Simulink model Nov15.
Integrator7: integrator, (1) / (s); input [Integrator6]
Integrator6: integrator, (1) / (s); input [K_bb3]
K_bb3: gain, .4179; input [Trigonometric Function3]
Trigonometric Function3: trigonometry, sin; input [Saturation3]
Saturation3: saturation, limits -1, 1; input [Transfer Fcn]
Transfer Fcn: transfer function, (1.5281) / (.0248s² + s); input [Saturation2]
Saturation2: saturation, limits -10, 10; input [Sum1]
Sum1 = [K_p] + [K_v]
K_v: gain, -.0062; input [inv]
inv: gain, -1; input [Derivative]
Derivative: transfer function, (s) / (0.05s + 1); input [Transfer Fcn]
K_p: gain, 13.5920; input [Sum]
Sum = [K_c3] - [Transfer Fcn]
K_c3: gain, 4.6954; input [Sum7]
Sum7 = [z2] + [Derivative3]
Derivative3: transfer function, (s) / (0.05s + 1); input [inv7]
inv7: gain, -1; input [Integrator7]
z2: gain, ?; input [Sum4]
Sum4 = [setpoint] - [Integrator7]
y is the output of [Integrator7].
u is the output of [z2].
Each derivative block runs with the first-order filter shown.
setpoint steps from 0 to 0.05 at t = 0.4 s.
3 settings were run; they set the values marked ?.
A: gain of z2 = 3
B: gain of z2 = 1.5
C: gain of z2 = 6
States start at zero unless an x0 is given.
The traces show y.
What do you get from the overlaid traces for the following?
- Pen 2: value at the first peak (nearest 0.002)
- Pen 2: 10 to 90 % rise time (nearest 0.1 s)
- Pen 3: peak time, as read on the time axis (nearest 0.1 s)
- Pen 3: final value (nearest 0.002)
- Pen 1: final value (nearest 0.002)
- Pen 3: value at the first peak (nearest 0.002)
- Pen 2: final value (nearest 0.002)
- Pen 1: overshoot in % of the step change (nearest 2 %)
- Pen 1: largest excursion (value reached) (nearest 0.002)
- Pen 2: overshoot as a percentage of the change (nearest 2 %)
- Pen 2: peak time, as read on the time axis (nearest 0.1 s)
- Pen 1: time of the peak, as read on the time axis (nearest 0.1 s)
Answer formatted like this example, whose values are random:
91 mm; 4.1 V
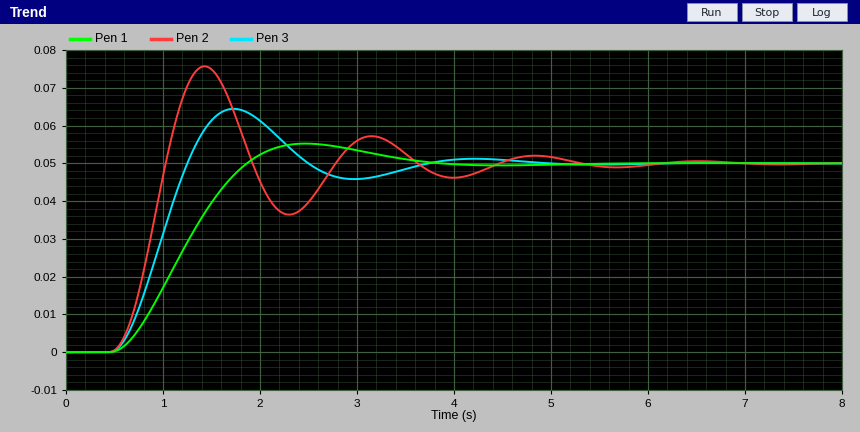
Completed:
0.076; 0.4 s; 1.7 s; 0.050; 0.050; 0.064; 0.050; 10 %; 0.056; 52 %; 1.4 s; 2.5 s
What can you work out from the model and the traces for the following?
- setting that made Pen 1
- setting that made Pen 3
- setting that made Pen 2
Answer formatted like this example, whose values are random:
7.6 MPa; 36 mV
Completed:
B; A; C
